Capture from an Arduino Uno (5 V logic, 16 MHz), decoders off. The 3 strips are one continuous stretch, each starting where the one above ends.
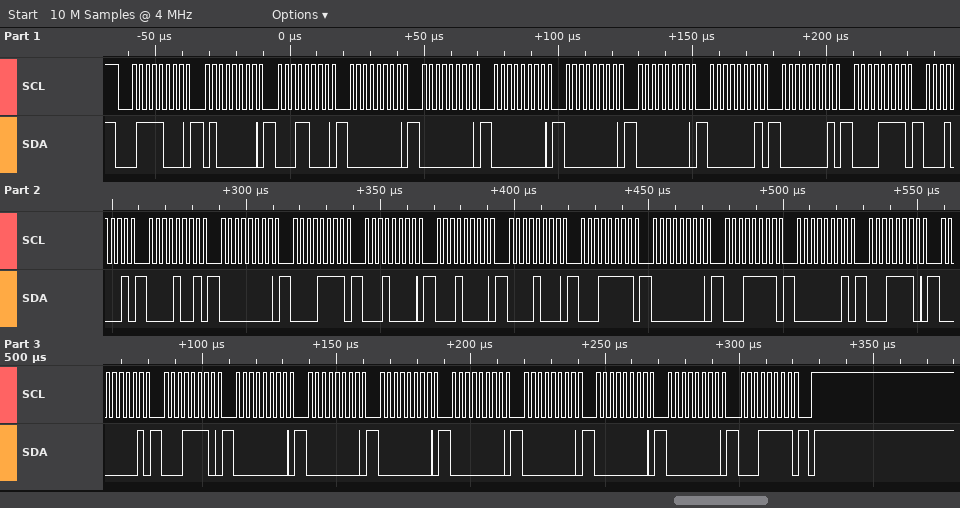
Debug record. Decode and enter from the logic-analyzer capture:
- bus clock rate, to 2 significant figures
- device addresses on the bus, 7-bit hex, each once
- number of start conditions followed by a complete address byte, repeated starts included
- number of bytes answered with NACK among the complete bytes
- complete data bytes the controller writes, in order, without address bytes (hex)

400 kHz
0x3C
1
0
40 18 00 00 00 00 00 01 01 0F 11 09 00 0F 10 10 08 1F 00 1F 01 1E 01 1E 00 00 00 00 00 00 00 1F
